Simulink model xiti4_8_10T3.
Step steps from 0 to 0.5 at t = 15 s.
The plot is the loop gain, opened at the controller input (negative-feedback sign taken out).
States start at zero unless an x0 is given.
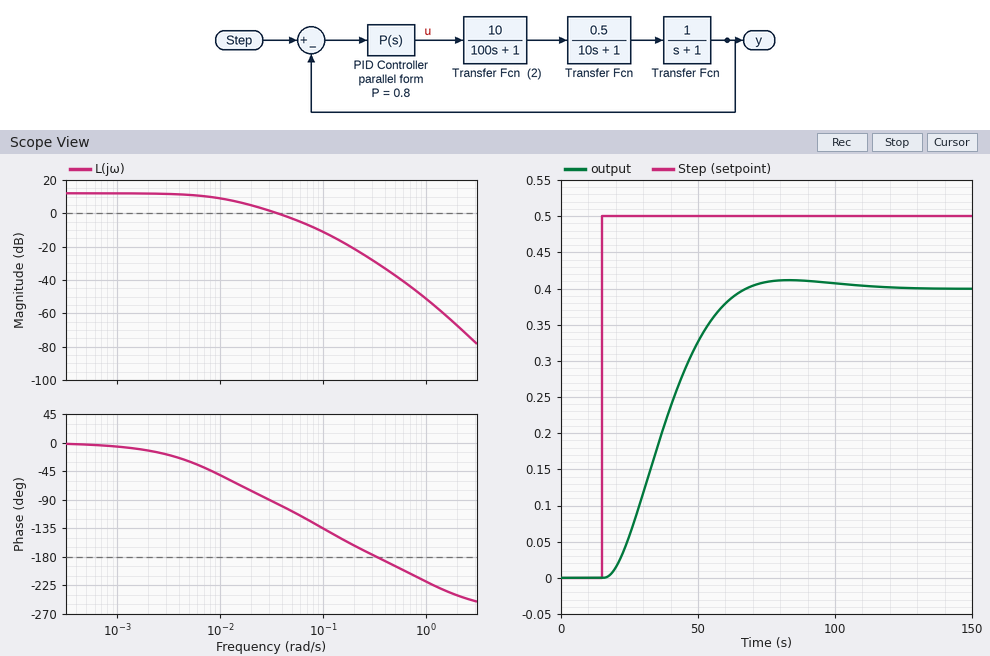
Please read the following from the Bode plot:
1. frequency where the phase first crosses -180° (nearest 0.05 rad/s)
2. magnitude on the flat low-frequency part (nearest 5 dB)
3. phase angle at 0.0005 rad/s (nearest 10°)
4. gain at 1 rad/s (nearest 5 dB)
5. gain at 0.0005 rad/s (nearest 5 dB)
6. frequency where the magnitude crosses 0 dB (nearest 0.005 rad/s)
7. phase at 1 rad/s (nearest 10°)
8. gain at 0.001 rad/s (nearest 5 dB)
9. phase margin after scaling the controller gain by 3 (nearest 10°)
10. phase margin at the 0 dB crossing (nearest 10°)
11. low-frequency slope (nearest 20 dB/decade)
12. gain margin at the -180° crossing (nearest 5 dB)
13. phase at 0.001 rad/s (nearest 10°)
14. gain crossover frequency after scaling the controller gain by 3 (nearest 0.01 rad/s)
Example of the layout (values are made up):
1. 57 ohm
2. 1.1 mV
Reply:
1. 0.35 rad/s
2. 10 dB
3. 0°
4. -50 dB
5. 10 dB
6. 0.035 rad/s
7. -220°
8. 10 dB
9. 50°
10. 80°
11. 0 dB/decade
12. 30 dB
13. -10°
14. 0.09 rad/s
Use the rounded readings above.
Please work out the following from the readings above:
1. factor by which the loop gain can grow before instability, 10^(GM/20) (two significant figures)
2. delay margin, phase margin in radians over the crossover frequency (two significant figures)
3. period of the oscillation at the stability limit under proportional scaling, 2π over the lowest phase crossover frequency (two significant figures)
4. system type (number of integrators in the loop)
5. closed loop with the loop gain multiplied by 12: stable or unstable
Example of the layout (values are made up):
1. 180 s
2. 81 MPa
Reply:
1. 32
2. 40 s
3. 18 s
4. 0
5. stable
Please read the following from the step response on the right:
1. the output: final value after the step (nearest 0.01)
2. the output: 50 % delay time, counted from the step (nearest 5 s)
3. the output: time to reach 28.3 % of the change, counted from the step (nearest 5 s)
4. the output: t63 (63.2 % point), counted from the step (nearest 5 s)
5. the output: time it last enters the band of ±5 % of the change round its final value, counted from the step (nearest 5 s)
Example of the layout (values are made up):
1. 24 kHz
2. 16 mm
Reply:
1. 0.40
2. 20 s
3. 15 s
4. 25 s
5. 45 s
